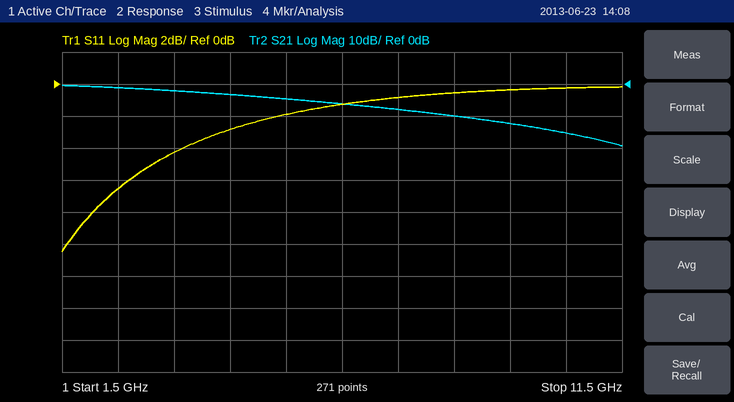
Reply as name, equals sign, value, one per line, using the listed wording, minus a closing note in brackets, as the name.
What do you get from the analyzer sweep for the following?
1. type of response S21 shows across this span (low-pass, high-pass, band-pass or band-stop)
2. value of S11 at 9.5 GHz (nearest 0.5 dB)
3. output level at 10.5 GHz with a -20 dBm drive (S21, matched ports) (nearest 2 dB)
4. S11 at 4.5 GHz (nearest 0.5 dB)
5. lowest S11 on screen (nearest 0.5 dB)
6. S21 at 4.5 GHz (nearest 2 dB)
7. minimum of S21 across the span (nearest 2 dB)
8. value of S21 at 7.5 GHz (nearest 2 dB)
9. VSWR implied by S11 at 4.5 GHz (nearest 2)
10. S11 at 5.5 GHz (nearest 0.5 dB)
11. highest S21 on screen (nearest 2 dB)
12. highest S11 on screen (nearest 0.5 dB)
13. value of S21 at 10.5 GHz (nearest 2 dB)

type of response S21 shows across this span = low-pass
value of S11 at 9.5 GHz = -0.5 dB
output level at 10.5 GHz with a -20 dBm drive (S21, matched ports) = -36 dBm
S11 at 4.5 GHz = -3.0 dB
lowest S11 on screen = -10.5 dB
S21 at 4.5 GHz = -4 dB
minimum of S21 across the span = -20 dB
value of S21 at 7.5 GHz = -8 dB
VSWR implied by S11 at 4.5 GHz = 6
S11 at 5.5 GHz = -2.0 dB
highest S21 on screen = 0 dB
highest S11 on screen = 0.0 dB
value of S21 at 10.5 GHz = -16 dB
